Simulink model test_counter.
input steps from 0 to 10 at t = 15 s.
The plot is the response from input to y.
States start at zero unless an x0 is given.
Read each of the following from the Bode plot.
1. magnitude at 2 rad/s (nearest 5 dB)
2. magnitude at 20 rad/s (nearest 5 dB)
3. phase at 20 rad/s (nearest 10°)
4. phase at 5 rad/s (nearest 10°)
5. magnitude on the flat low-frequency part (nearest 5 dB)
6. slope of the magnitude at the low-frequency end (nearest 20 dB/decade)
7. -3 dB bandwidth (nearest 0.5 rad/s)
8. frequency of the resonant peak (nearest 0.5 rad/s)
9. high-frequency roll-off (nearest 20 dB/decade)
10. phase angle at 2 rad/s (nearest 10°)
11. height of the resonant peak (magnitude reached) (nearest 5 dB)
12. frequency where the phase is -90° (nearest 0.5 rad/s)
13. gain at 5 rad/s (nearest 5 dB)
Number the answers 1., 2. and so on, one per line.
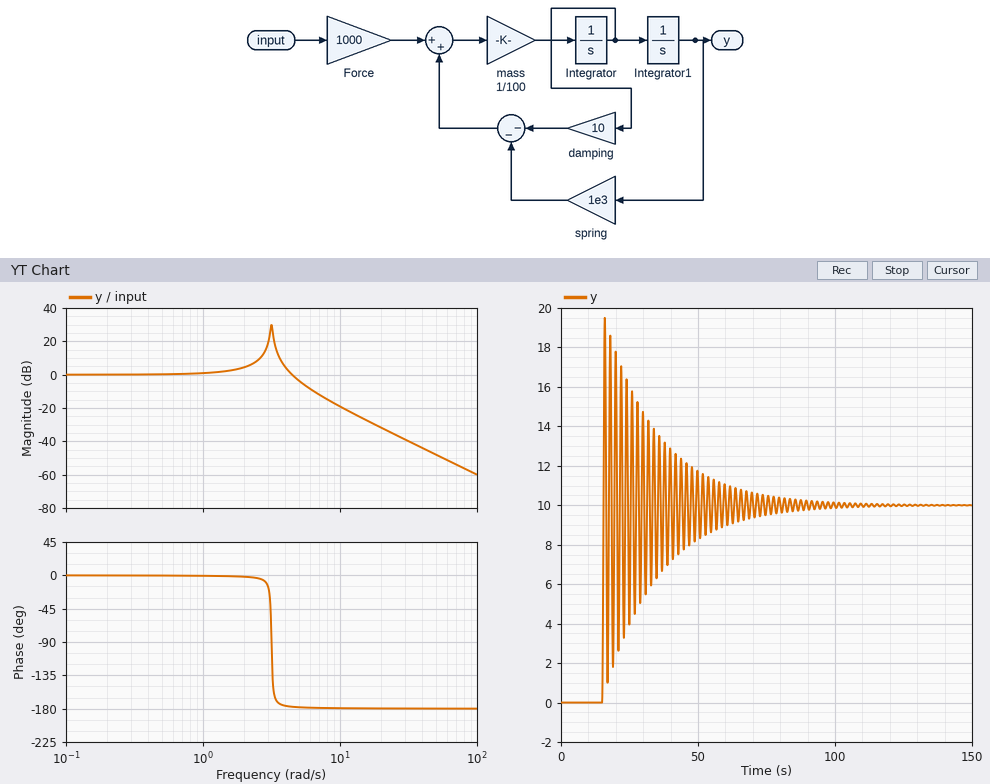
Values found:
1. 5 dB
2. -30 dB
3. -180°
4. -180°
5. 0 dB
6. 0 dB/decade
7. 5.0 rad/s
8. 3.0 rad/s
9. -40 dB/decade
10. 0°
11. 30 dB
12. 3.0 rad/s
13. -5 dB
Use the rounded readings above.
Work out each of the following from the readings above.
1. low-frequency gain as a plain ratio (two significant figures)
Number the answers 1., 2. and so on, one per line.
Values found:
1. 1.0
